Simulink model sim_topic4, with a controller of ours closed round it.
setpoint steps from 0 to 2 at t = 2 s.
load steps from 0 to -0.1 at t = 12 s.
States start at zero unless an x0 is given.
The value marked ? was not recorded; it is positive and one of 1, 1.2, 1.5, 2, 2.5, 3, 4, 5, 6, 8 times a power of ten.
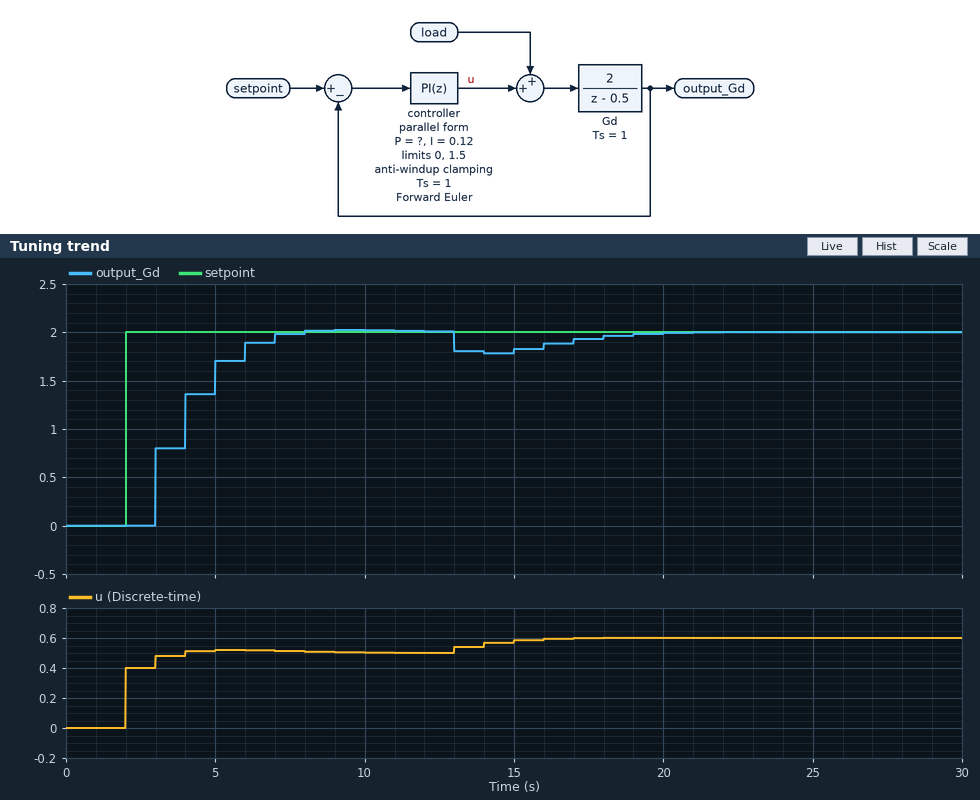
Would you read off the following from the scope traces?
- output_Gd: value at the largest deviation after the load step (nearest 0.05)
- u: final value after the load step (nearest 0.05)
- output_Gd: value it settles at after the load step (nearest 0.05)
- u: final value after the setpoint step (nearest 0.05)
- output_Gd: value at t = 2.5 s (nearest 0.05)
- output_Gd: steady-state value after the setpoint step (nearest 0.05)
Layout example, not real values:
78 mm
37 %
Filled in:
1.80
0.60
2.00
0.50
0.00
2.00
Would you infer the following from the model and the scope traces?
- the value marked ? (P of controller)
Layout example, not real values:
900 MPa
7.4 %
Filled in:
0.2
